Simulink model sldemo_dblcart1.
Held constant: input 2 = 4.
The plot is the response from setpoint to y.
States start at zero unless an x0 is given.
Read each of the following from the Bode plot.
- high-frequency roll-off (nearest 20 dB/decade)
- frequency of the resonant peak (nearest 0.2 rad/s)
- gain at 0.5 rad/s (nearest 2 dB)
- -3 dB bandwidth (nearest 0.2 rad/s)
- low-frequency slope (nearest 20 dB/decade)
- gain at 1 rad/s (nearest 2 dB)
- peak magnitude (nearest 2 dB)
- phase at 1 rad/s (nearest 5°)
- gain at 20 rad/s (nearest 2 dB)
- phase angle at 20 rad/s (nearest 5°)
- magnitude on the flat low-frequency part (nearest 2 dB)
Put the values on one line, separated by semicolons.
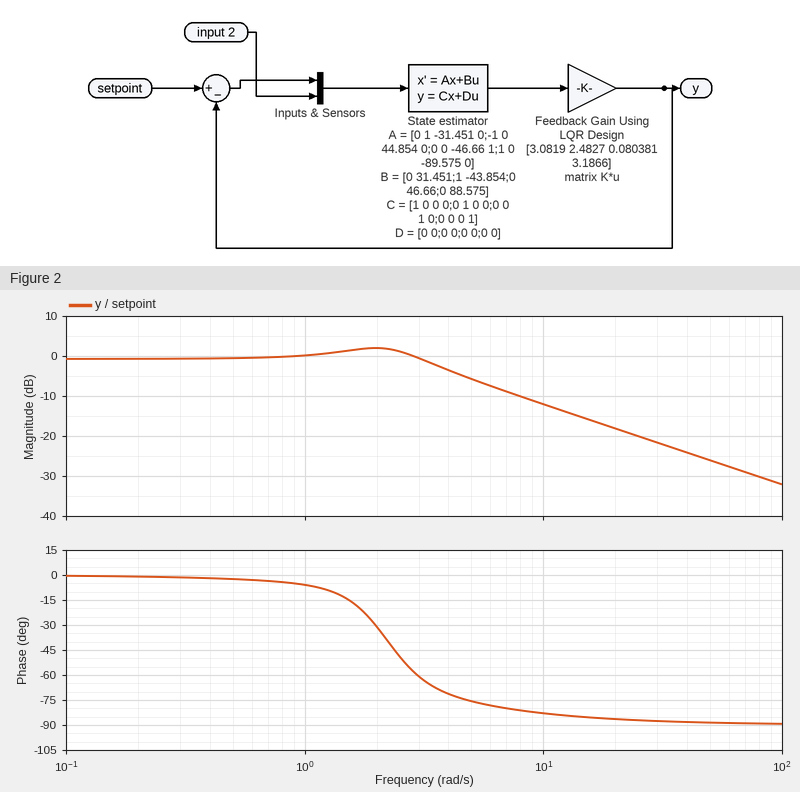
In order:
-20 dB/decade; 2.0 rad/s; 0 dB; 4.0 rad/s; 0 dB/decade; 0 dB; 2 dB; -5°; -18 dB; -85°; 0 dB
